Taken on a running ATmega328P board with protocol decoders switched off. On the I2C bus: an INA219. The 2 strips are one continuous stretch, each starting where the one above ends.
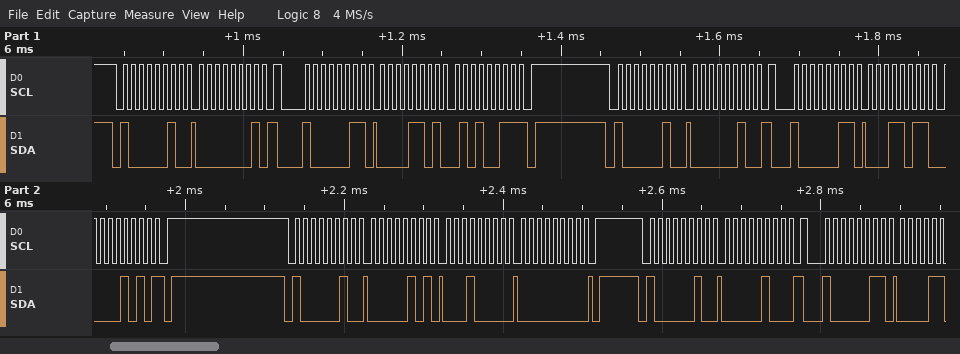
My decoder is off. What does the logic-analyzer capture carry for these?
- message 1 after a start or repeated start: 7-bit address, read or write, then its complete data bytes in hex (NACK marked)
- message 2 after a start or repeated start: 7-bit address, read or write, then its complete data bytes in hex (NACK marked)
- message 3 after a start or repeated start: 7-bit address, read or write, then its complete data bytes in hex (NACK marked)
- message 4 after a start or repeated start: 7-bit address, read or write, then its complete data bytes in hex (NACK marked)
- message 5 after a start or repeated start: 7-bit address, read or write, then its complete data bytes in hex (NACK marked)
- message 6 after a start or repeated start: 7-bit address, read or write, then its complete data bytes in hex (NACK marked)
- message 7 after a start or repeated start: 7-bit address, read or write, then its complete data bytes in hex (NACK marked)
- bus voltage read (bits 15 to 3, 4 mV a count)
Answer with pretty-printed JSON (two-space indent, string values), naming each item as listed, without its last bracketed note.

{
  "message 1 after a start or repeated start: 7-bit address, read or write, then its complete data bytes in hex": "0x41 write: 01",
  "message 2 after a start or repeated start: 7-bit address, read or write, then its complete data bytes in hex": "0x41 read: 0D 53 NACK",
  "message 3 after a start or repeated start: 7-bit address, read or write, then its complete data bytes in hex": "0x41 write: 02",
  "message 4 after a start or repeated start: 7-bit address, read or write, then its complete data bytes in hex": "0x41 read: 1B 0A NACK",
  "message 5 after a start or repeated start: 7-bit address, read or write, then its complete data bytes in hex": "0x41 write: 05 10 00",
  "message 6 after a start or repeated start: 7-bit address, read or write, then its complete data bytes in hex": "0x41 write: 04",
  "message 7 after a start or repeated start: 7-bit address, read or write, then its complete data bytes in hex": "0x41 read",
  "bus voltage read": "3.460 V"
}
